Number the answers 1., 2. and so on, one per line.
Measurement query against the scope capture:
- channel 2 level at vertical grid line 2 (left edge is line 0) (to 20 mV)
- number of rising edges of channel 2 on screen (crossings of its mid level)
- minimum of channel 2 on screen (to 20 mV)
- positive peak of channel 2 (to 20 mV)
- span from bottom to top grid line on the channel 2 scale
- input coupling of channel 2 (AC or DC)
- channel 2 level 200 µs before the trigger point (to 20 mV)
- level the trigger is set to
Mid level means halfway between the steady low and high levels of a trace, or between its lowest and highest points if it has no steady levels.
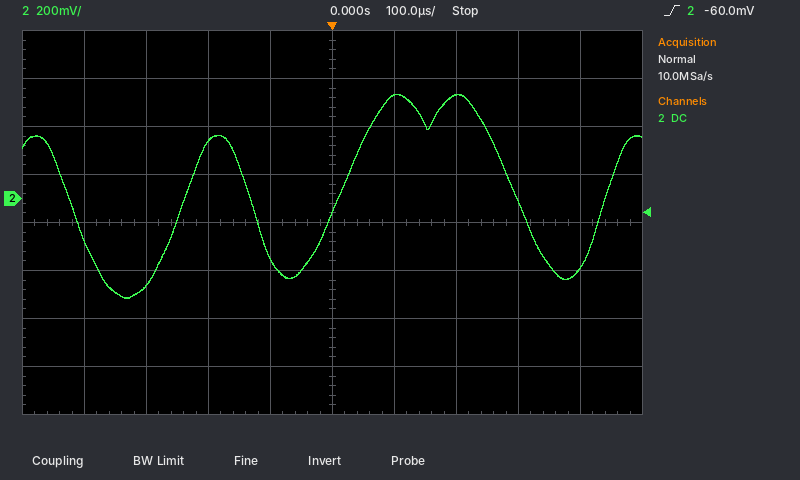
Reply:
1. -360 mV
2. 3
3. -420 mV
4. 440 mV
5. 1.6 V
6. DC
7. 240 mV
8. -60.0 mV
